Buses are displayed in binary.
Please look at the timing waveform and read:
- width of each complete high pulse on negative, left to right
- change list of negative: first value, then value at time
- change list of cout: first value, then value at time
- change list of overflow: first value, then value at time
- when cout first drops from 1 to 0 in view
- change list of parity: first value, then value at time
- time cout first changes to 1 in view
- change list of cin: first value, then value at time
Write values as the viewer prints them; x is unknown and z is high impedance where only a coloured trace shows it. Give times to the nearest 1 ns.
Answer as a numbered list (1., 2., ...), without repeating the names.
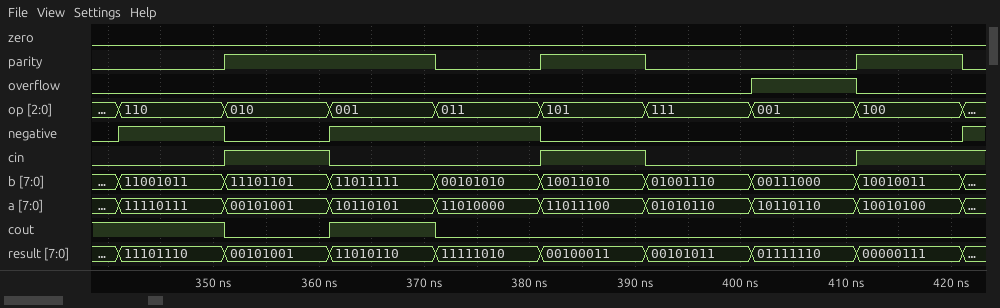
1. 10 ns, 20 ns
2. 0, 1 at 341 ns, 0 at 351 ns, 1 at 361 ns, 0 at 381 ns, 1 at 421 ns
3. 1, 0 at 351 ns, 1 at 361 ns, 0 at 371 ns
4. 0, 1 at 401 ns, 0 at 411 ns
5. 351 ns
6. 0, 1 at 351 ns, 0 at 371 ns, 1 at 381 ns, 0 at 391 ns, 1 at 411 ns, 0 at 421 ns
7. 361 ns
8. 0, 1 at 351 ns, 0 at 361 ns, 1 at 381 ns, 0 at 391 ns, 1 at 411 ns
